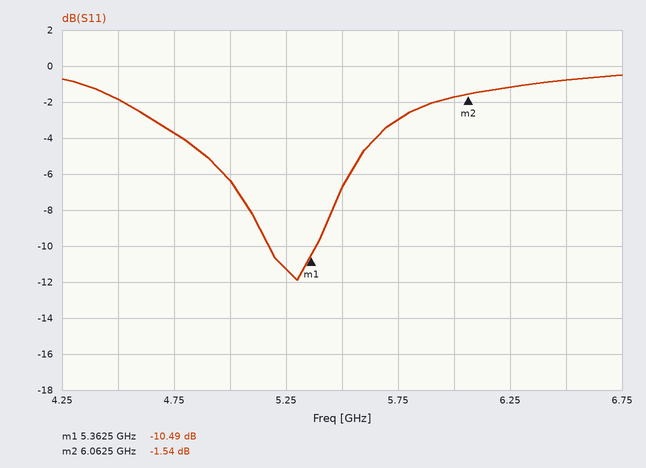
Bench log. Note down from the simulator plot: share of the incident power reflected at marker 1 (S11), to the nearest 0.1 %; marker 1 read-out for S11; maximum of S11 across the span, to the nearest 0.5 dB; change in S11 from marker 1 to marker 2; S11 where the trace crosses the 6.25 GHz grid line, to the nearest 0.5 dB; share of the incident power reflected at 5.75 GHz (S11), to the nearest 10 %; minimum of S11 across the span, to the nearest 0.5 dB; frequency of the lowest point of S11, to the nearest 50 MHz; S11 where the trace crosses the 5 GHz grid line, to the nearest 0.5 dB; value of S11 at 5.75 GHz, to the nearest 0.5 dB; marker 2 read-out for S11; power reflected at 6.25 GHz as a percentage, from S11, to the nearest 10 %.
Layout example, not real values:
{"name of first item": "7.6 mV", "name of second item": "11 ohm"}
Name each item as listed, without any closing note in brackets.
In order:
{"share of the incident power reflected at marker 1 (S11), to the nearest 0.1 %": "8.9 %", "marker 1 read-out for S11": "-10.49 dB", "maximum of S11 across the span, to the nearest 0.5 dB": "-0.5 dB", "change in S11 from marker 1 to marker 2": "8.95 dB", "S11 where the trace crosses the 6.25 GHz grid line, to the nearest 0.5 dB": "-1.0 dB", "share of the incident power reflected at 5.75 GHz (S11), to the nearest 10 %": "50 %", "minimum of S11 across the span, to the nearest 0.5 dB": "-12.0 dB", "frequency of the lowest point of S11, to the nearest 50 MHz": "5.30 GHz", "S11 where the trace crosses the 5 GHz grid line, to the nearest 0.5 dB": "-6.5 dB", "value of S11 at 5.75 GHz, to the nearest 0.5 dB": "-3.0 dB", "marker 2 read-out for S11": "-1.54 dB", "power reflected at 6.25 GHz as a percentage, from S11, to the nearest 10 %": "80 %"}
